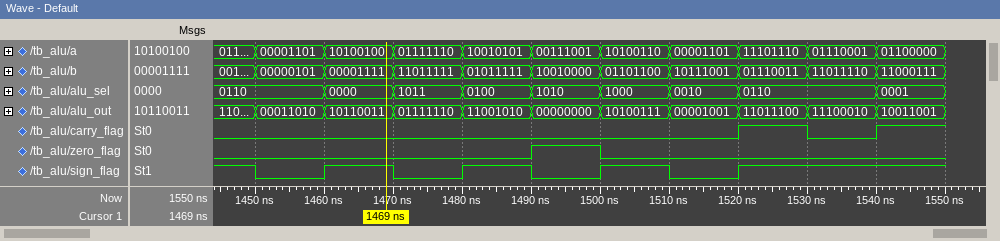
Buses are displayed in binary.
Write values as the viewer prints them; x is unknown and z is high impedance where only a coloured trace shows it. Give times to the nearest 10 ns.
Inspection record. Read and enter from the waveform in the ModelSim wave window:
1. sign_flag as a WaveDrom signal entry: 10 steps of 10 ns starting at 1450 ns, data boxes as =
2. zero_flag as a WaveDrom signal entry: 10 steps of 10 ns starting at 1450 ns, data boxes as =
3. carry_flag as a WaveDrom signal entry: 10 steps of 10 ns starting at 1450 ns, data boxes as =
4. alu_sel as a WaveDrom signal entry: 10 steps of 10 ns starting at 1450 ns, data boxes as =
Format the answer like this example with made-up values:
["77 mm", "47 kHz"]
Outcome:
["{name: 'sign_flag', wave: '01010101..'}", "{name: 'zero_flag', wave: '0...10....'}", "{name: 'carry_flag', wave: '0......101'}", "{name: 'alu_sel', wave: '========.=', data: '0110 0000 1011 0100 1010 1000 0010 0110 0001'}"]
